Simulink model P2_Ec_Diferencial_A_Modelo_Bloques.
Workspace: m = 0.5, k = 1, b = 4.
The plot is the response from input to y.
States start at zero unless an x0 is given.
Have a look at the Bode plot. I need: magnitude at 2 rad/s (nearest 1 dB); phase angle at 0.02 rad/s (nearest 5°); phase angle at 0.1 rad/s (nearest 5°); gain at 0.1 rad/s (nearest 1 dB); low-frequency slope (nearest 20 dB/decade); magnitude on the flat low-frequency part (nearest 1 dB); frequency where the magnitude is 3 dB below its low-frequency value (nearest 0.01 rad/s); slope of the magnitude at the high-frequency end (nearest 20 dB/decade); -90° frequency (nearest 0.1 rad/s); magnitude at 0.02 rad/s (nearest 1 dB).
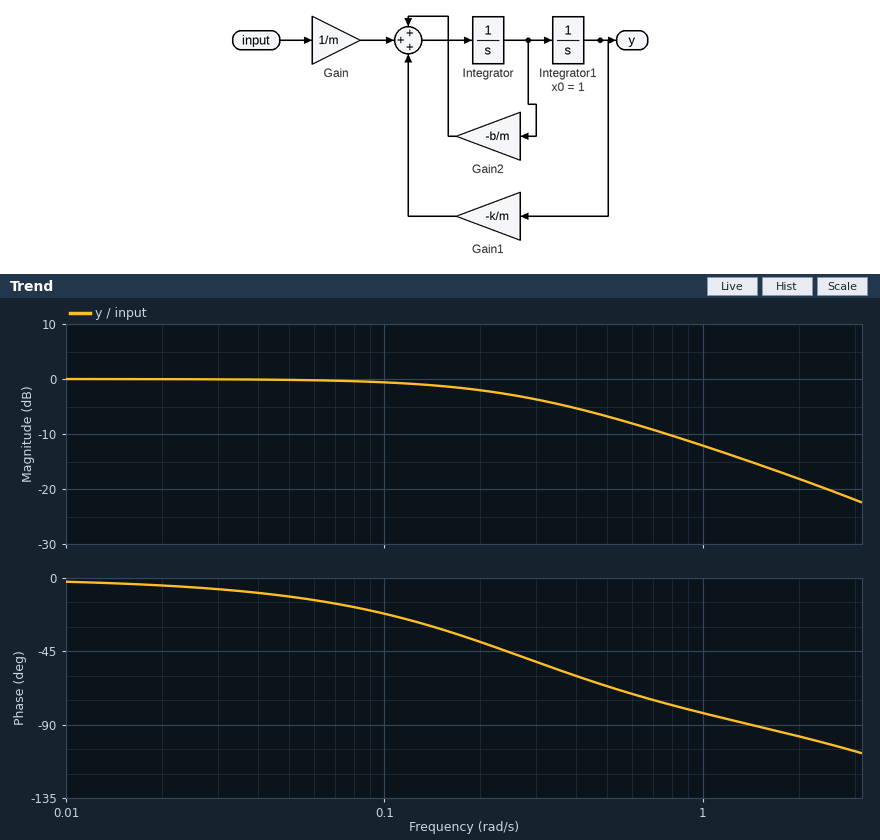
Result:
-18 dB
-5°
-20°
-1 dB
0 dB/decade
0 dB
0.26 rad/s
-20 dB/decade
1.4 rad/s
0 dB
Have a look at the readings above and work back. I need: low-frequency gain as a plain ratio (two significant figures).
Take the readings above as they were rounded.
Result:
1.0
